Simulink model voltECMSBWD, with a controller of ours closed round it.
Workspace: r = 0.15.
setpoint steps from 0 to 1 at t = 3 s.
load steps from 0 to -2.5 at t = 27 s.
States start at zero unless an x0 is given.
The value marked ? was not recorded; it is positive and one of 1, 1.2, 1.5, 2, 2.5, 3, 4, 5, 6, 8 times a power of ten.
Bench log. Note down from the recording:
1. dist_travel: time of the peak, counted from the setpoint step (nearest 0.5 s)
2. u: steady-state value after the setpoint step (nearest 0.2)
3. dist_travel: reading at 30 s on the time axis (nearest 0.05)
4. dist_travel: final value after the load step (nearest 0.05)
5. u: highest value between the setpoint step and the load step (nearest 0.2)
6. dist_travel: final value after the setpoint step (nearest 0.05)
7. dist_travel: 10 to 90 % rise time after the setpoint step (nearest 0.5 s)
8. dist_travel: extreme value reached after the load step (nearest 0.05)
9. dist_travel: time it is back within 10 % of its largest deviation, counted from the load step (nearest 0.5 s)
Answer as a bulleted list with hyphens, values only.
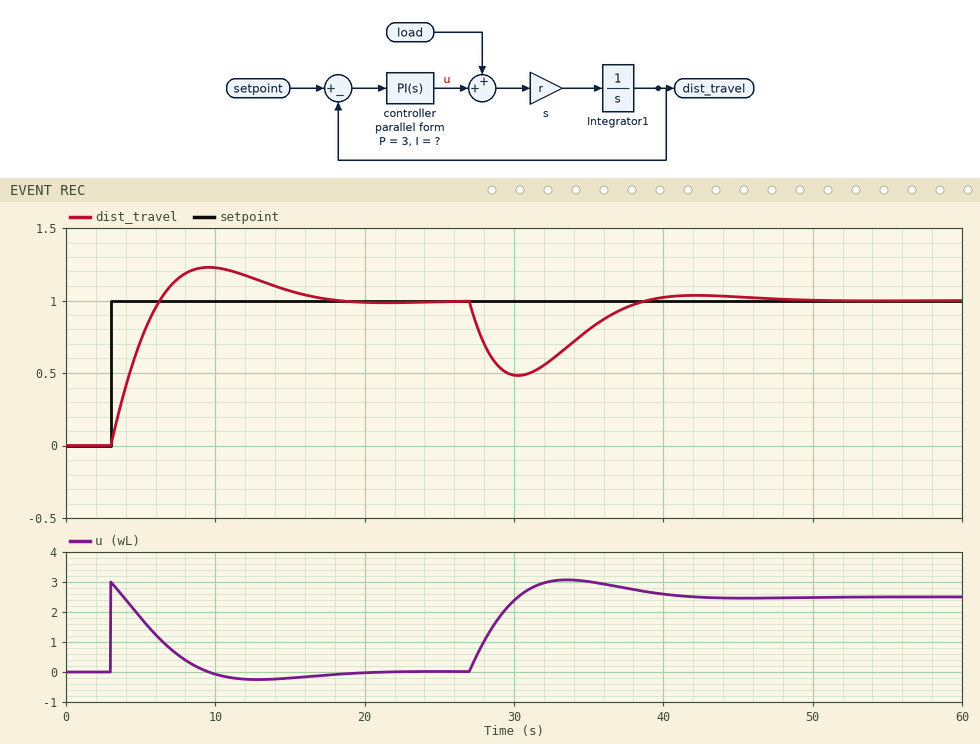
- 6.5 s
- 0.0
- 0.50
- 1.00
- 3.0
- 1.00
- 2.5 s
- 0.50
- 10.5 s
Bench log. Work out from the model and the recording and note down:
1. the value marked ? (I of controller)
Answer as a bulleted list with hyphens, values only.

- 0.8
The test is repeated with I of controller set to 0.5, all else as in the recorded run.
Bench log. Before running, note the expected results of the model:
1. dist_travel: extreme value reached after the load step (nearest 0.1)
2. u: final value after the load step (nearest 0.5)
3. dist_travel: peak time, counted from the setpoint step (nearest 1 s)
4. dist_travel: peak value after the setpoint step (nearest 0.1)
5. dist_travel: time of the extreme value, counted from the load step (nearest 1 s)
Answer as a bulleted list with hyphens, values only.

- 0.4
- 2.5
- 8 s
- 1.2
- 4 s
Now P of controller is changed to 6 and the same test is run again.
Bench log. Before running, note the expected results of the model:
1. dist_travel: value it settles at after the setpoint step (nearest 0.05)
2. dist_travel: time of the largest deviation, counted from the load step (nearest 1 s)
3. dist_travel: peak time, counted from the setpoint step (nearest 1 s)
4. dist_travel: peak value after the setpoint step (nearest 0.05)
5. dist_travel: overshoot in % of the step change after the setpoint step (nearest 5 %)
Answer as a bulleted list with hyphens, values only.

- 1.00
- 3 s
- 5 s
- 1.10
- 10 %
